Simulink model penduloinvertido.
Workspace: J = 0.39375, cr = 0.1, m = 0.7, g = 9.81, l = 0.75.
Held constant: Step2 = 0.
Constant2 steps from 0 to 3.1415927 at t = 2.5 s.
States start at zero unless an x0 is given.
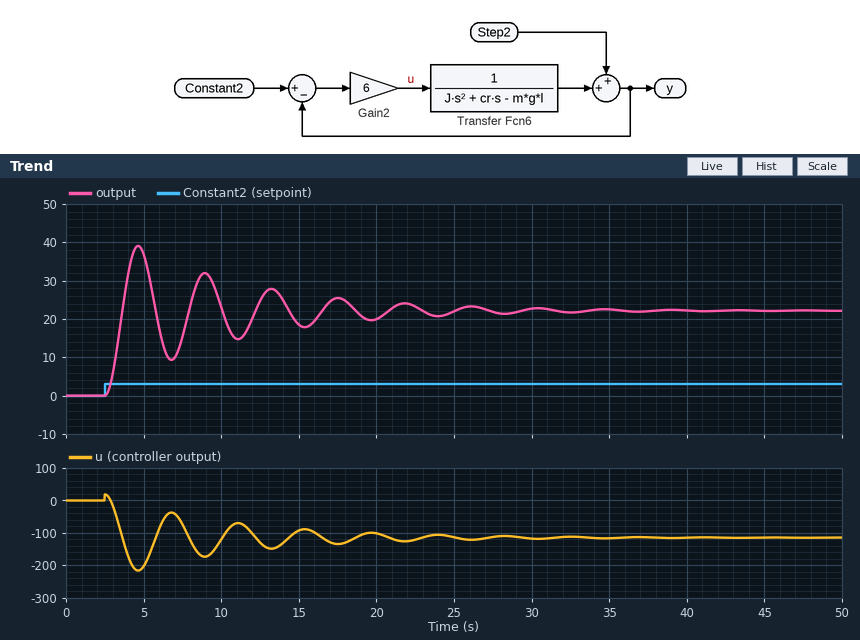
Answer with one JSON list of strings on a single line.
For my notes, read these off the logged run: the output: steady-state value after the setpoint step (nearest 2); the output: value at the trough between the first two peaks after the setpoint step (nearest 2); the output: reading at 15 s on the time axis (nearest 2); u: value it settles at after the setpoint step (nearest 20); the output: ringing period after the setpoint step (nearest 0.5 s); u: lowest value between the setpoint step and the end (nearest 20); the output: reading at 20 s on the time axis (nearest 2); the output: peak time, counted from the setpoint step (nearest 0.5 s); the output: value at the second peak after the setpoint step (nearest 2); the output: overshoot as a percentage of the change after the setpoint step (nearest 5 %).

["22", "10", "18", "-120", "4.5 s", "-220", "20", "2.0 s", "32", "75 %"]
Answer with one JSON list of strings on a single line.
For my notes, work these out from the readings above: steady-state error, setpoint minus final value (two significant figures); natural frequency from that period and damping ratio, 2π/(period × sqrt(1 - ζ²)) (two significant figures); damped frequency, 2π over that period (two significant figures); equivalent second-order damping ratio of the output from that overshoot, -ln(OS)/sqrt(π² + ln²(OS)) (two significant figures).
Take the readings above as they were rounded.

["-19", "1.4 rad/s", "1.4 rad/s", "0.091"]
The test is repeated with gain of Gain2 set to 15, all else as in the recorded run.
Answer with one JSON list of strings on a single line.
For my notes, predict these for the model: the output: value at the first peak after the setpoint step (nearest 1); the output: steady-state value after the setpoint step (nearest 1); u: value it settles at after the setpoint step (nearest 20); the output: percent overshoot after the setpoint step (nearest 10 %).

["9", "5", "-20", "90 %"]
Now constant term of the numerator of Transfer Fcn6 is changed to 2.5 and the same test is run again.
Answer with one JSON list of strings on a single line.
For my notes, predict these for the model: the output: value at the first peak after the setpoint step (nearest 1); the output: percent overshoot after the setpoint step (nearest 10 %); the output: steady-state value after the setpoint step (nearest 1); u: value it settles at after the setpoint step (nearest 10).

["9", "90 %", "5", "-10"]
